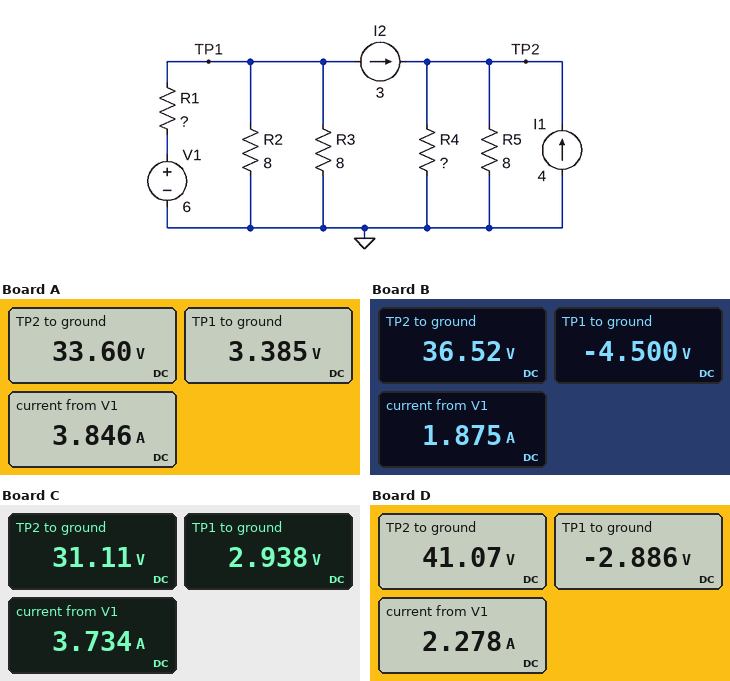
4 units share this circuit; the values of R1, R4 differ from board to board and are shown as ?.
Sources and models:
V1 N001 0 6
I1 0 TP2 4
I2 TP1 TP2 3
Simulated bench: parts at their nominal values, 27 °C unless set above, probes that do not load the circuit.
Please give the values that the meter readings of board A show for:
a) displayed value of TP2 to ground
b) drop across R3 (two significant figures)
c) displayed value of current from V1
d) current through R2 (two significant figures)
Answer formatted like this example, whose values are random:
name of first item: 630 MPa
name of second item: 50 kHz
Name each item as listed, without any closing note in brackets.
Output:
displayed value of TP2 to ground: 33.60 V
drop across R3: 3.4 V
displayed value of current from V1: 3.846 A
current through R2: 420 mA
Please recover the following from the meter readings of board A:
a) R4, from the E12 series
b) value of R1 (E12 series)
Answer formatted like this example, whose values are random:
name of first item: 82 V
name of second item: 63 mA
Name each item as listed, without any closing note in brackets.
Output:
R4, from the E12 series: 12 Ω
value of R1: 0.68 Ω
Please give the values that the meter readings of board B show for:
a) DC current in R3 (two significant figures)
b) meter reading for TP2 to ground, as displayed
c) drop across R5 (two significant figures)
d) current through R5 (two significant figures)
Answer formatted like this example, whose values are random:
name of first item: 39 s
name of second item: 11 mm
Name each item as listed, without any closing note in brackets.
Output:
DC current in R3: 560 mA
meter reading for TP2 to ground, as displayed: 36.52 V
drop across R5: 37 V
current through R5: 4.6 A
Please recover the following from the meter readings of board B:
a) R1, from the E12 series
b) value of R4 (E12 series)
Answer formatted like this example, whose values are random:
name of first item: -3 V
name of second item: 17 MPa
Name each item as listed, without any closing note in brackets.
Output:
R1, from the E12 series: 5.6 Ω
value of R4: 15 Ω
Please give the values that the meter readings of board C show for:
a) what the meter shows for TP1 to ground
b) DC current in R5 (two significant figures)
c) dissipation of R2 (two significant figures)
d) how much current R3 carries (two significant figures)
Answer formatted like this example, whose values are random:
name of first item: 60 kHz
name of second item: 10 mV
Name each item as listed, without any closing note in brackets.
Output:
what the meter shows for TP1 to ground: 2.938 V
DC current in R5: 3.9 A
dissipation of R2: 1.1 W
how much current R3 carries: 370 mA
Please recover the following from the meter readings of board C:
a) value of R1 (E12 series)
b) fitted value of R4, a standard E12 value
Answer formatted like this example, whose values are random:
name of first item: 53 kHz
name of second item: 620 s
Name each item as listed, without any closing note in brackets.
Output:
value of R1: 0.82 Ω
fitted value of R4, a standard E12 value: 10 Ω
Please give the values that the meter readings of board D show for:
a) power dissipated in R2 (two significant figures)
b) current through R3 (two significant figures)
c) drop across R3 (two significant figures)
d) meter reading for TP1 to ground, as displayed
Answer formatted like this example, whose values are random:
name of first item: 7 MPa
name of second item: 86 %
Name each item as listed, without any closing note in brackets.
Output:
power dissipated in R2: 1.0 W
current through R3: 360 mA
drop across R3: 2.9 V
meter reading for TP1 to ground, as displayed: -2.886 V
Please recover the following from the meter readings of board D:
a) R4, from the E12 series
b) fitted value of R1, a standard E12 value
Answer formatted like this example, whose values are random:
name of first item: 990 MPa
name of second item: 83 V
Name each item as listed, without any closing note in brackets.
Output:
R4, from the E12 series: 22 Ω
fitted value of R1, a standard E12 value: 3.9 Ω
